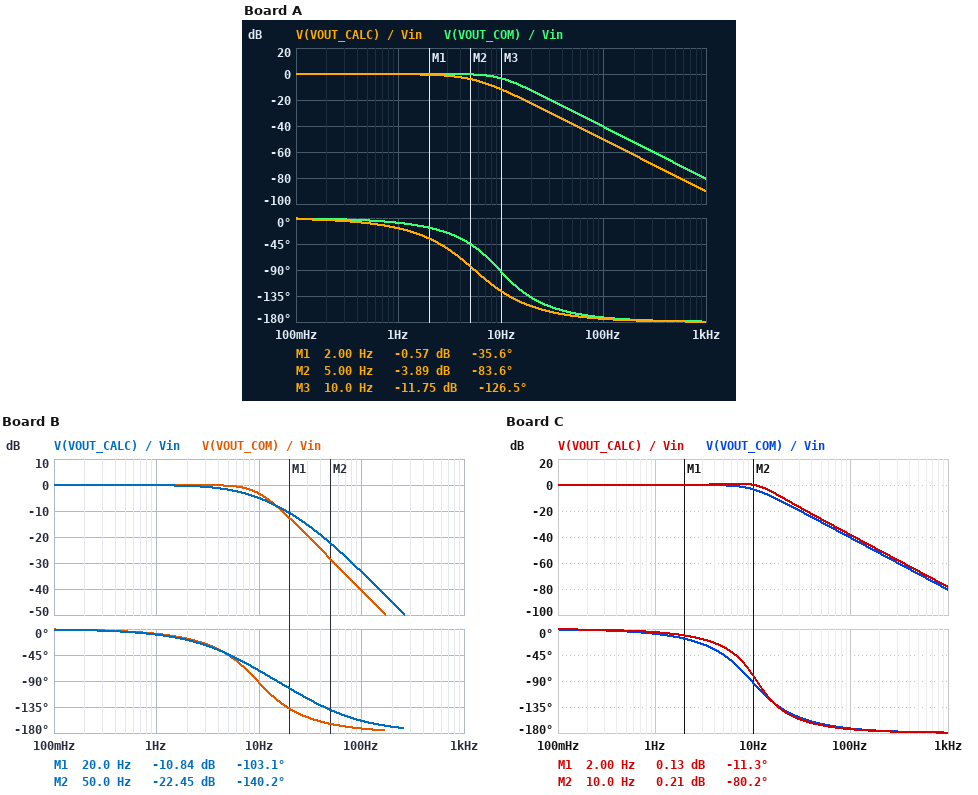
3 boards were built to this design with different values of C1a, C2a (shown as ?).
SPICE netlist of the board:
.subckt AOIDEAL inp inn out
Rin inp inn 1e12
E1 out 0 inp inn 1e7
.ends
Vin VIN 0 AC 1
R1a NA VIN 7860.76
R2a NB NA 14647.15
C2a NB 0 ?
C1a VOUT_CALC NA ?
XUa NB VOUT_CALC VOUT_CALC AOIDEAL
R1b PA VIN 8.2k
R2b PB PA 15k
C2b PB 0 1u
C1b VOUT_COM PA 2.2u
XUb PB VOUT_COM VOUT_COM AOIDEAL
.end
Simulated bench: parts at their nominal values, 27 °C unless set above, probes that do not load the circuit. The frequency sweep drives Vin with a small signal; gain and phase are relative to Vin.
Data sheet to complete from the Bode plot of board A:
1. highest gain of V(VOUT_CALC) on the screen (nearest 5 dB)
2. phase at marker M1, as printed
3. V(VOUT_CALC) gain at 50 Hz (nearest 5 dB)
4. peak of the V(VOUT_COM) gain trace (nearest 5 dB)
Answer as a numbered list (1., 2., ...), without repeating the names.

1. 0 dB
2. -35.6 deg
3. -40 dB
4. 0 dB
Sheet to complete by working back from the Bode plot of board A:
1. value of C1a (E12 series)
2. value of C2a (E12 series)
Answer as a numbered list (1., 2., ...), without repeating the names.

1. 3.3 µF
2. 2.2 µF
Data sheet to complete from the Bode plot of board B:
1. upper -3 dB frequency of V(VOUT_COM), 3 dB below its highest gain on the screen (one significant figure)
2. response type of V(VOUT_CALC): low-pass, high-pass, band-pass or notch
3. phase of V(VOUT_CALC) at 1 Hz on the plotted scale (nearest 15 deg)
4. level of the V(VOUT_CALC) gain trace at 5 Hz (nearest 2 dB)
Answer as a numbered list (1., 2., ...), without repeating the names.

1. 10 Hz
2. low-pass
3. -15 deg
4. -2 dB
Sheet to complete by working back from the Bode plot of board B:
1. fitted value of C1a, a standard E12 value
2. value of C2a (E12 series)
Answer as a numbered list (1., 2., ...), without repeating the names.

1. 820 nF
2. 1.2 µF
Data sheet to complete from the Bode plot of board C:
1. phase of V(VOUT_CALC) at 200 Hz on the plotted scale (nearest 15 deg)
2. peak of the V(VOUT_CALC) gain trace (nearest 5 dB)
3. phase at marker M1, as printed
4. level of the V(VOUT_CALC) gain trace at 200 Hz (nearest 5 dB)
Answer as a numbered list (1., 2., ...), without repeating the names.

1. -180 deg
2. 0 dB
3. -11.3 deg
4. -50 dB
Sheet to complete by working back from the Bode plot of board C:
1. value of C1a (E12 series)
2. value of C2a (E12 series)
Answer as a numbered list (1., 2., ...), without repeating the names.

1. 2.7 µF
2. 680 nF
